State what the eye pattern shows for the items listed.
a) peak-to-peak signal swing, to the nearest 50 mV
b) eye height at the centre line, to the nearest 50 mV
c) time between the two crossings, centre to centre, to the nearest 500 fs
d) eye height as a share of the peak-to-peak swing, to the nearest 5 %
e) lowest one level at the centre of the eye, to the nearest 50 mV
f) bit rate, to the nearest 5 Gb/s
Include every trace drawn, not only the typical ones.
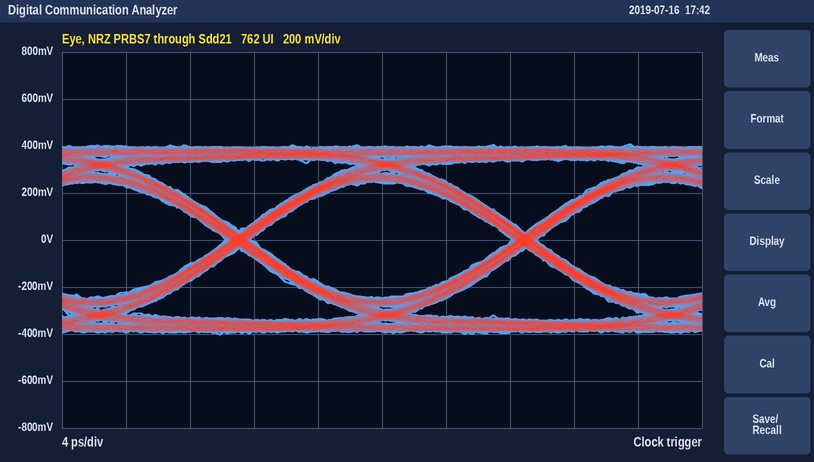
800 mV
500 mV
18.0 ps
60 %
250 mV
55 Gb/s
